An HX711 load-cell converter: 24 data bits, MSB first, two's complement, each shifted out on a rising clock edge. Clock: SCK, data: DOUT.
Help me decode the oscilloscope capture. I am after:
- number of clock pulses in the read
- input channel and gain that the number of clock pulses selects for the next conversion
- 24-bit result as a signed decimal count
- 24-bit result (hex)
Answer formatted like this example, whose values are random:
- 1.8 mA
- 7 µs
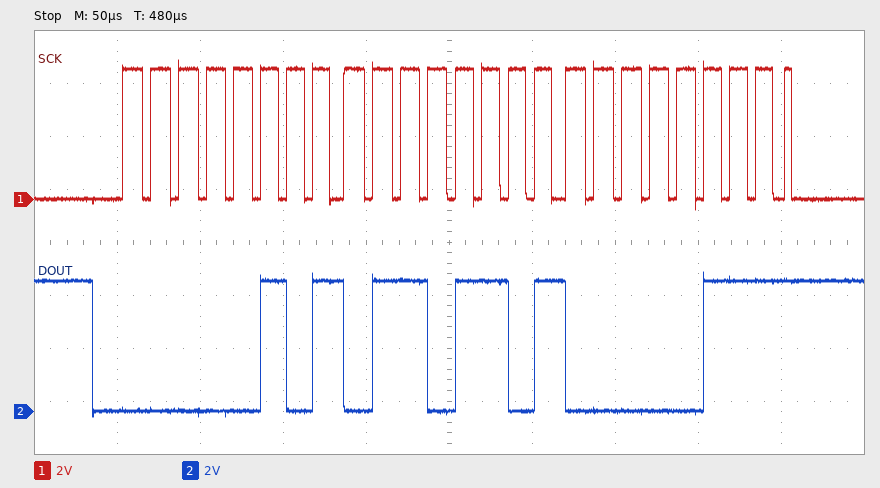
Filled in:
- 25
- channel A, gain 128
- 355591
- 0x056D07
